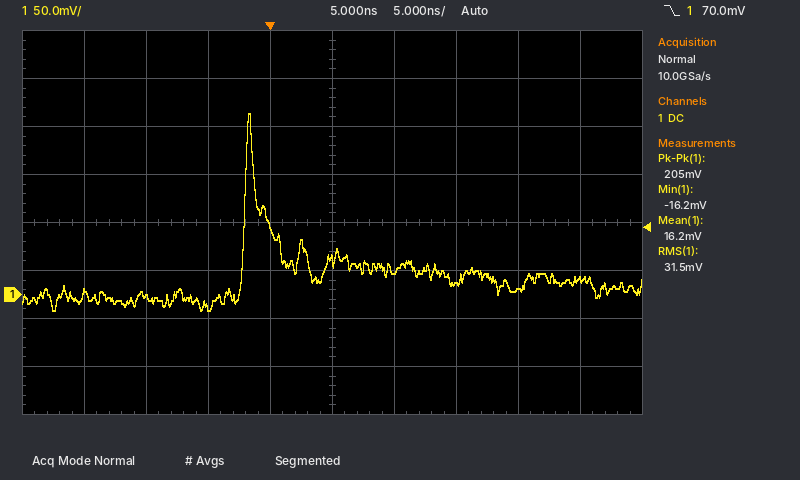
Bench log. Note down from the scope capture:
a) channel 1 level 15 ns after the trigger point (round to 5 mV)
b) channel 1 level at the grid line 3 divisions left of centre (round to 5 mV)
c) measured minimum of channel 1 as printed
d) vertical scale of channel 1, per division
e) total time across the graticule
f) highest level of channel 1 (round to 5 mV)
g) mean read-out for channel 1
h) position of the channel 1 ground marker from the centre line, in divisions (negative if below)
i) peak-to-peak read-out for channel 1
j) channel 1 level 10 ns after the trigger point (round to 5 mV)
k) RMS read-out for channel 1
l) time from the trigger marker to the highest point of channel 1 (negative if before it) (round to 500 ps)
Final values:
10 mV
-5 mV
-16.2 mV
50 mV
50 ns
190 mV
16.2 mV
-1.5 div
205 mV
25 mV
31.5 mV
-1.5 ns
